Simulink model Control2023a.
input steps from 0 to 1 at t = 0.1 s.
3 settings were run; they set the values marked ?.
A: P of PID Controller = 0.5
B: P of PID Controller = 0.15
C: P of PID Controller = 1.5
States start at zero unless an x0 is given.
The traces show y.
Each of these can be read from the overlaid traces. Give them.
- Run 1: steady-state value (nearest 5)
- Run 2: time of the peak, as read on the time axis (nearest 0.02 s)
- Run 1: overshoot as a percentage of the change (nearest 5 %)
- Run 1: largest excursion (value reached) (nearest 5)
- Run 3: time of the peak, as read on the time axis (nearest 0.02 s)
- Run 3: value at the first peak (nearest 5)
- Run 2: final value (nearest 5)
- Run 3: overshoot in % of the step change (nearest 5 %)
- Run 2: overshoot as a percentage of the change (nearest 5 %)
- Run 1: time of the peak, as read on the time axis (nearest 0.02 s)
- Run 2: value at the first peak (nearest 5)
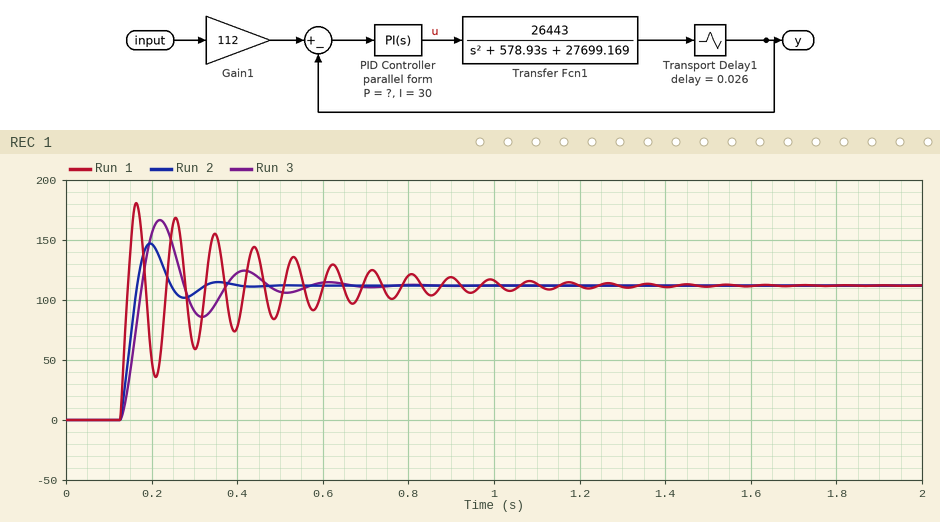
110
0.20 s
60 %
180
0.22 s
165
110
50 %
30 %
0.16 s
145
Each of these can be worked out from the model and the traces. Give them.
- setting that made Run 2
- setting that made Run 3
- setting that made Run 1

A
B
C
